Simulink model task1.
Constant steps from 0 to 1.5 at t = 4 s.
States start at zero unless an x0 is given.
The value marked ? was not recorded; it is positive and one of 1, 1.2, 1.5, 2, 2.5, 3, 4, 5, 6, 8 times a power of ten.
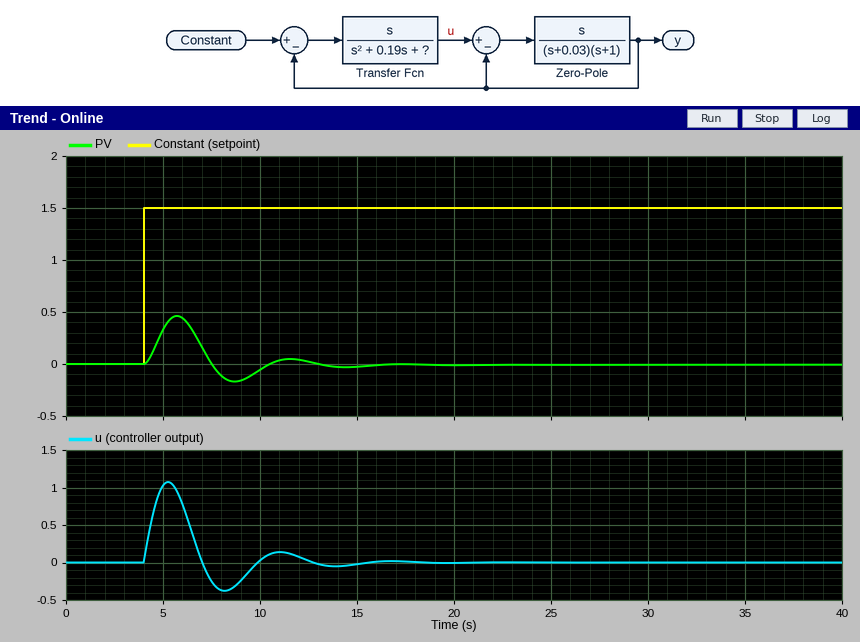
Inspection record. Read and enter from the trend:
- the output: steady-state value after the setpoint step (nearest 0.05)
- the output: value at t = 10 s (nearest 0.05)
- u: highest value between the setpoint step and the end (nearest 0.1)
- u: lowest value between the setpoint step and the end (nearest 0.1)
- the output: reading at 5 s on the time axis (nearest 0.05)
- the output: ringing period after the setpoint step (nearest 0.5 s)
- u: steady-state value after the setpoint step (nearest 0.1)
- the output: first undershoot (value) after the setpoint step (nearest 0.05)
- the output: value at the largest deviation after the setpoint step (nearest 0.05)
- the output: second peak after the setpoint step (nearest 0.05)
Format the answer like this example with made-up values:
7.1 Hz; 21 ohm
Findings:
0.00; -0.05; 1.1; -0.4; 0.35; 6.0 s; 0.0; -0.15; 0.45; 0.05
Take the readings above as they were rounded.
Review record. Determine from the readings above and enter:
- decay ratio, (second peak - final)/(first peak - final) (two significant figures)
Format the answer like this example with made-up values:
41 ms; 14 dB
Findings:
0.11
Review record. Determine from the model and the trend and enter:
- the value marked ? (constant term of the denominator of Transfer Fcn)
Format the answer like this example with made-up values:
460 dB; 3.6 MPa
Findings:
1
